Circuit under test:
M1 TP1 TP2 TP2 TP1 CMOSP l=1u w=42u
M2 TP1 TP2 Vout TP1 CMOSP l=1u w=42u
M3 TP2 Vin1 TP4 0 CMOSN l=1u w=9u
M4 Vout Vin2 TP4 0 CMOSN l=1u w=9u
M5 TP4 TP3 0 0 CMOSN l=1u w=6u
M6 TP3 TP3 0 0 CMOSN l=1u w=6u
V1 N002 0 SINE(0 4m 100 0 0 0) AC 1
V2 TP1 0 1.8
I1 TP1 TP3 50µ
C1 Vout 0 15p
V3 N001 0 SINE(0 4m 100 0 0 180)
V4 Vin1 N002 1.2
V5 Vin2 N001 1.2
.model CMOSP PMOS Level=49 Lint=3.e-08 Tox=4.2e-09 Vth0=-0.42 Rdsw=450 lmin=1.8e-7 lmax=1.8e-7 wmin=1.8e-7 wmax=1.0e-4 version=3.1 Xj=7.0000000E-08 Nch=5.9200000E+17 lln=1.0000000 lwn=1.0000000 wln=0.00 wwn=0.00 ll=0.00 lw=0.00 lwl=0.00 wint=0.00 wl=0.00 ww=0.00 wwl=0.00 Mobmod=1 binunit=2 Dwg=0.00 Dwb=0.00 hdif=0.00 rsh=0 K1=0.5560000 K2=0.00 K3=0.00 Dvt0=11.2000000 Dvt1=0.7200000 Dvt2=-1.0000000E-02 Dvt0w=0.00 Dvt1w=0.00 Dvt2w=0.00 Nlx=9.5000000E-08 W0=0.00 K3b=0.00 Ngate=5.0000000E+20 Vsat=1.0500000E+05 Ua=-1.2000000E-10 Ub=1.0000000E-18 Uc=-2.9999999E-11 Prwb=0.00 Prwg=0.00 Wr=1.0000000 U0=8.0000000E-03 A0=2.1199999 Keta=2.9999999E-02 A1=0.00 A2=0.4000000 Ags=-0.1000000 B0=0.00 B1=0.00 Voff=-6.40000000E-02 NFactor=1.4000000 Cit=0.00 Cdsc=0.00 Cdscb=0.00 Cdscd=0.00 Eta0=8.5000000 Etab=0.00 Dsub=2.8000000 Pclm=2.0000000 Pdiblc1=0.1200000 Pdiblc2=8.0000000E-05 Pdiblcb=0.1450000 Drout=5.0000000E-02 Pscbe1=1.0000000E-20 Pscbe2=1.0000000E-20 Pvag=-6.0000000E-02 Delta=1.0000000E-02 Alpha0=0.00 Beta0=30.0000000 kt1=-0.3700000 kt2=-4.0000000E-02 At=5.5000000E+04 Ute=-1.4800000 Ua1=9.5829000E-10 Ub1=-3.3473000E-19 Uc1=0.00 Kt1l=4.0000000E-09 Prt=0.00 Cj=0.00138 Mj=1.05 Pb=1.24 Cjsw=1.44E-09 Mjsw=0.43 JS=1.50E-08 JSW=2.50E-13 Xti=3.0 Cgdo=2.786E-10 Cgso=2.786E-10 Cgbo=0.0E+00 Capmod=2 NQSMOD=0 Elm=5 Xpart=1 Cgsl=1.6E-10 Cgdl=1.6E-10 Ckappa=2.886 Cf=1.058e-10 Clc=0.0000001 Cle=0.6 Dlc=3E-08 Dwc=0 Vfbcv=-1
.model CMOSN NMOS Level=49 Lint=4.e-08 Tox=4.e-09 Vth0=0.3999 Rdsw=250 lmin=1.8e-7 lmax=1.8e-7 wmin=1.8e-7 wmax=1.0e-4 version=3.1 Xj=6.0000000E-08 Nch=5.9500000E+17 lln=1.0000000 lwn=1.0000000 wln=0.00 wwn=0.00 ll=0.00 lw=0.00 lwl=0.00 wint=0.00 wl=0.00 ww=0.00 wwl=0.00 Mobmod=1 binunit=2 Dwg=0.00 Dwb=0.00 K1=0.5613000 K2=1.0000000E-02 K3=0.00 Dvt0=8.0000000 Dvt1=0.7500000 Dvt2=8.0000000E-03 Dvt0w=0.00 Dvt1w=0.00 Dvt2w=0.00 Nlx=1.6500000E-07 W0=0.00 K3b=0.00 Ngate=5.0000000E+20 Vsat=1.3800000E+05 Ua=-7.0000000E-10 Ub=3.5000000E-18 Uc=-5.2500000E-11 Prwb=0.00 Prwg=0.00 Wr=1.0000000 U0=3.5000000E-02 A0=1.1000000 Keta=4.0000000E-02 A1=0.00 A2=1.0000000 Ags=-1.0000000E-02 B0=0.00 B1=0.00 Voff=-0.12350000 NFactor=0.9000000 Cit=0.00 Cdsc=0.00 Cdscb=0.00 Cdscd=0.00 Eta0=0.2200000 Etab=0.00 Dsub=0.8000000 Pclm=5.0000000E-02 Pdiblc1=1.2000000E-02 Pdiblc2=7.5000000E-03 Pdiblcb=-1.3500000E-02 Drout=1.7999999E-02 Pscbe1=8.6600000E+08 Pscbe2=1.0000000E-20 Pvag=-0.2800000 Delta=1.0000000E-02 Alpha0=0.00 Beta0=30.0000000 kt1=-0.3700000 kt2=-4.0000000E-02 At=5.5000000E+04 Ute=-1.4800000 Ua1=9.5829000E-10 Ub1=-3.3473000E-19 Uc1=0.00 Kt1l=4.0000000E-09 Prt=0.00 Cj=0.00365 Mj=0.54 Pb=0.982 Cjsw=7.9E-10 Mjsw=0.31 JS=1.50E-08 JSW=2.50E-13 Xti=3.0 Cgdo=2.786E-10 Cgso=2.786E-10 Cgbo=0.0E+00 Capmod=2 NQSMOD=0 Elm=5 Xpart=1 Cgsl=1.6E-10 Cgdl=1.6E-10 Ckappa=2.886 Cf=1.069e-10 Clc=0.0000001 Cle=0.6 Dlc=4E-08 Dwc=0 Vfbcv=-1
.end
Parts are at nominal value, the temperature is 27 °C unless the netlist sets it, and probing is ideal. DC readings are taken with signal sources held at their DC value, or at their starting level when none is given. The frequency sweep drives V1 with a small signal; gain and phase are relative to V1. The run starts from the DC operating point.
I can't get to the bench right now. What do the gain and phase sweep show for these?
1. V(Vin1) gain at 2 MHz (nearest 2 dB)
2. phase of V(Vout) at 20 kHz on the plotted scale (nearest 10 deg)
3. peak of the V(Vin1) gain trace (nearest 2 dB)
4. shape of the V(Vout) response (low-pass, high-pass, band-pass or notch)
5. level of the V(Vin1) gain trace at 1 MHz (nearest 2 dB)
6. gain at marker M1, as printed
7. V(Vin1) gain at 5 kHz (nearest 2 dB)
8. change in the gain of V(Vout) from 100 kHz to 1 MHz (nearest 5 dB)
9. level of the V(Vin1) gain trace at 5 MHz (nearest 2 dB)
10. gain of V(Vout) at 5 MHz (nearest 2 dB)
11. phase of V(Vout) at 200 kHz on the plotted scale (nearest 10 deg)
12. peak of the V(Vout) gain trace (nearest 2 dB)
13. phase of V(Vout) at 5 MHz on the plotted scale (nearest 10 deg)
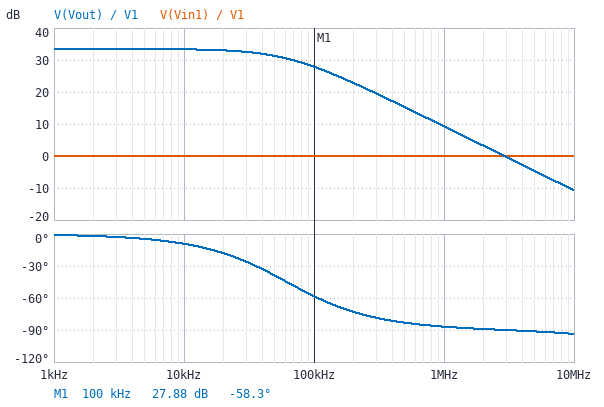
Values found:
0 dB
-20 deg
0 dB
low-pass
0 dB
27.88 dB
0 dB
-20 dB
0 dB
-4 dB
-70 deg
34 dB
-90 deg
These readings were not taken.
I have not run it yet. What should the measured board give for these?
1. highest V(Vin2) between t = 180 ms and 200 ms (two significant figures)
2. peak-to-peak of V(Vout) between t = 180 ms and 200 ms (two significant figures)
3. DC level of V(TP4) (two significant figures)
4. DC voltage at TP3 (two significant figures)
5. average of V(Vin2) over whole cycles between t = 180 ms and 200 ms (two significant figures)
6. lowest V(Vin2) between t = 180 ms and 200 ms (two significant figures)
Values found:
1.2 V
730 mV
490 mV
690 mV
1.2 V
1.2 V
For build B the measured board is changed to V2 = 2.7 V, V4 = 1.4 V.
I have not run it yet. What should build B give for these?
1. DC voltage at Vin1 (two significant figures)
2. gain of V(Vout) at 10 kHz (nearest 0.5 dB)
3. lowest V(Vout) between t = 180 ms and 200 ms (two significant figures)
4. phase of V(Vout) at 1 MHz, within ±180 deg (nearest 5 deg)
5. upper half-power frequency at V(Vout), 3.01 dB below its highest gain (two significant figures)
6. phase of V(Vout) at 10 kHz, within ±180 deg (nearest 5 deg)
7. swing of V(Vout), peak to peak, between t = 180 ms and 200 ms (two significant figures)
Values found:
1.4 V
-19.0 dB
2.7 V
-10 deg
5.1 MHz
0 deg
1.8 mV
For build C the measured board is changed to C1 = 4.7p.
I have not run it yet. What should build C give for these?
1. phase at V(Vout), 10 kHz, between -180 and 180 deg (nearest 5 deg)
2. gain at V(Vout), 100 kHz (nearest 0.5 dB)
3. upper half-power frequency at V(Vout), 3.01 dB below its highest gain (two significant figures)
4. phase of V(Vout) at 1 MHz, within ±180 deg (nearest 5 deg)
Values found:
-5 deg
32.5 dB
190 kHz
-80 deg
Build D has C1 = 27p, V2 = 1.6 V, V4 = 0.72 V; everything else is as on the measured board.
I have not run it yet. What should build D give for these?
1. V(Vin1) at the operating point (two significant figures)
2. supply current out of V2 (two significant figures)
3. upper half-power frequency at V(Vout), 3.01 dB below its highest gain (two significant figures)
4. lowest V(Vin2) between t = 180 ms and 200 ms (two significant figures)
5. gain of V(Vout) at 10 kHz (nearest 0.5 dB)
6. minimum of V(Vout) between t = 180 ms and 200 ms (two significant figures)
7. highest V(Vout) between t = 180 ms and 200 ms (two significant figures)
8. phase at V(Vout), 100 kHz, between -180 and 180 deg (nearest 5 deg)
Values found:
720 mV
89 µA
3.4 MHz
1.2 V
-3.5 dB
150 mV
160 mV
0 deg
